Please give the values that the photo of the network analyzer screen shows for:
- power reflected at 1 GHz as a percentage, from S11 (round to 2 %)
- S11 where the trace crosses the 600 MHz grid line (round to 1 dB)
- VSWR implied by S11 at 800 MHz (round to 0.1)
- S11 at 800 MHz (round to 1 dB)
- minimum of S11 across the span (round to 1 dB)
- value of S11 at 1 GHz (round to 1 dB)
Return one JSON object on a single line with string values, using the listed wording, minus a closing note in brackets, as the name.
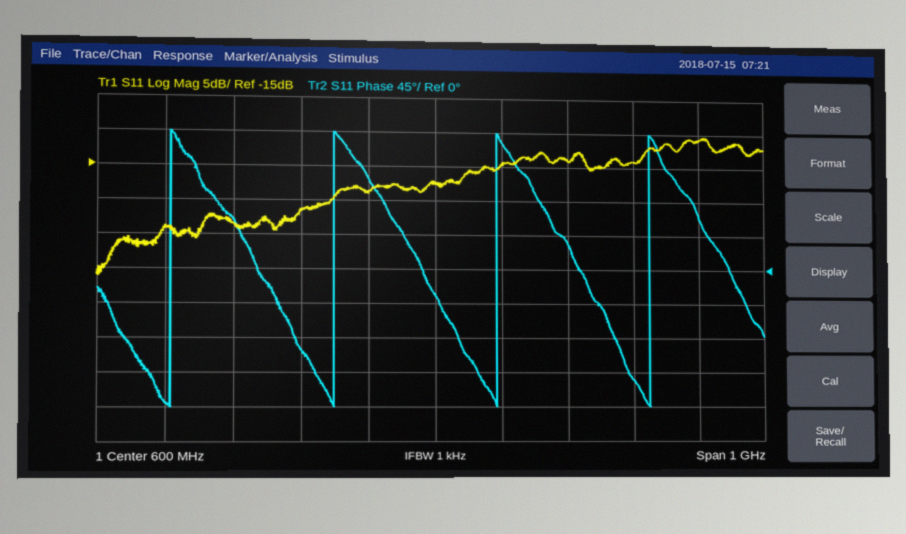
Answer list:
{"power reflected at 1 GHz as a percentage, from S11": "8 %", "S11 where the trace crosses the 600 MHz grid line": "-17 dB", "VSWR implied by S11 at 800 MHz": "1.5", "S11 at 800 MHz": "-14 dB", "minimum of S11 across the span": "-31 dB", "value of S11 at 1 GHz": "-11 dB"}
